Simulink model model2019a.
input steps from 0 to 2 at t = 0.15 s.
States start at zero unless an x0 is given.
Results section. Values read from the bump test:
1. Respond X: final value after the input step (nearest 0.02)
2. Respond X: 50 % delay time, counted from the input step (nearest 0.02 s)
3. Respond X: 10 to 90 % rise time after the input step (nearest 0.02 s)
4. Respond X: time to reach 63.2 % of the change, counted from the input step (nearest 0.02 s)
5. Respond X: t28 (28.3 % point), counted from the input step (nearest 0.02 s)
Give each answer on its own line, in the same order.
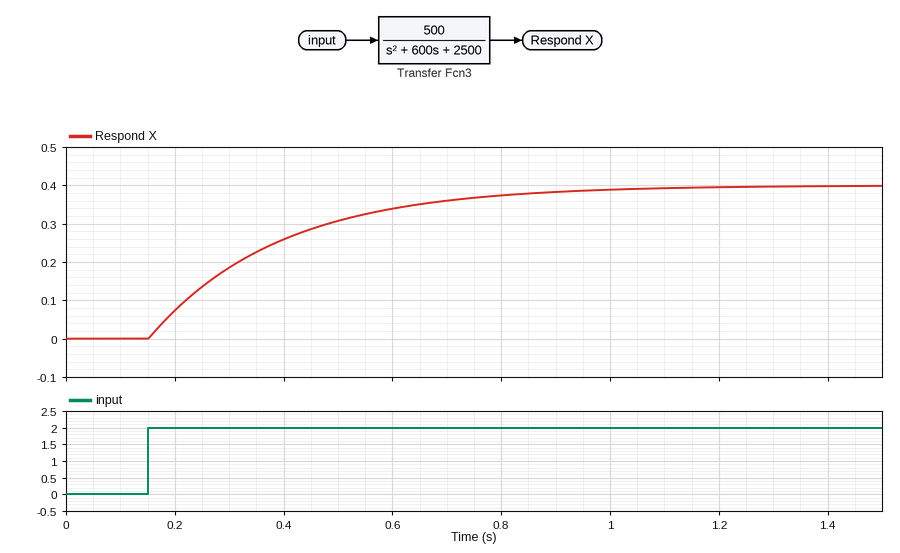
0.40
0.16 s
0.52 s
0.24 s
0.08 s
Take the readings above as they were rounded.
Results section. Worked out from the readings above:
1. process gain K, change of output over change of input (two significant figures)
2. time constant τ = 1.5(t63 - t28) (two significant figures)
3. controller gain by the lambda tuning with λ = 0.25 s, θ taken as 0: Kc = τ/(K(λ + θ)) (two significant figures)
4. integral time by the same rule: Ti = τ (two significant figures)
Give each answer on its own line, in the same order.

0.20
0.24 s
4.8
0.24 s
